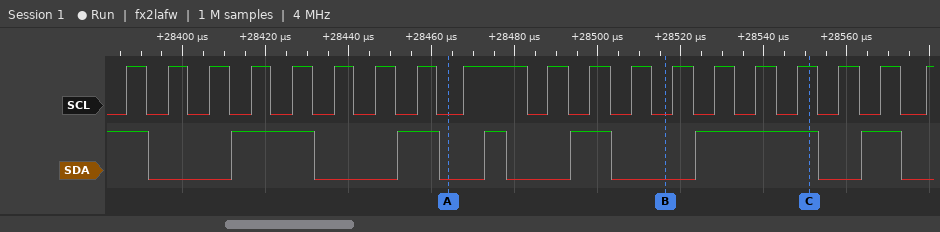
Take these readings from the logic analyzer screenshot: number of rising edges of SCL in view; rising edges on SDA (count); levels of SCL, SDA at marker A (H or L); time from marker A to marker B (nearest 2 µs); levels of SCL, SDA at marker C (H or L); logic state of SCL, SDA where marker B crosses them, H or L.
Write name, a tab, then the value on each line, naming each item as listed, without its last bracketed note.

number of rising edges of SCL in view	19
rising edges on SDA	6
levels of SCL, SDA at marker A	SCL=L, SDA=L
time from marker A to marker B	52 µs
levels of SCL, SDA at marker C	SCL=H, SDA=H
logic state of SCL, SDA where marker B crosses them, H or L	SCL=L, SDA=L
